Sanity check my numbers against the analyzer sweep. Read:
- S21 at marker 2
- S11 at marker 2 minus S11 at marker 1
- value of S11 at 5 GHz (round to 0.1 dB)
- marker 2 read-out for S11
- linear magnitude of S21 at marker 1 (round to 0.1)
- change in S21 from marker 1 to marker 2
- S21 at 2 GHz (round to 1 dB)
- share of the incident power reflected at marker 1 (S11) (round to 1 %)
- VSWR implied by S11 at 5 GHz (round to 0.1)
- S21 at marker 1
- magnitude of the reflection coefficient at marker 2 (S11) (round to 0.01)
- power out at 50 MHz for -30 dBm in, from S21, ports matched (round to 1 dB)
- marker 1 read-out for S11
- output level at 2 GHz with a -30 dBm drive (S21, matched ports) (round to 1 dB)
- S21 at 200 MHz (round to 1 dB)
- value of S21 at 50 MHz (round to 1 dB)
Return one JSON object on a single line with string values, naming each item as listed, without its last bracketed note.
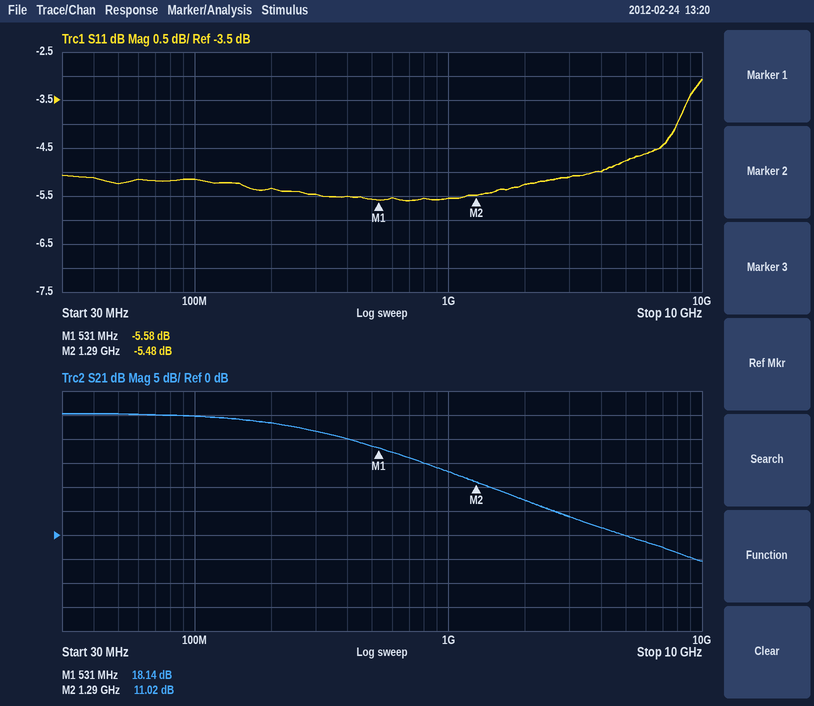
{"S21 at marker 2": "11.02 dB", "S11 at marker 2 minus S11 at marker 1": "0.10 dB", "value of S11 at 5 GHz": "-4.8 dB", "marker 2 read-out for S11": "-5.48 dB", "linear magnitude of S21 at marker 1": "8.1", "change in S21 from marker 1 to marker 2": "-7.12 dB", "S21 at 2 GHz": "7 dB", "share of the incident power reflected at marker 1 (S11)": "28 %", "VSWR implied by S11 at 5 GHz": "3.7", "S21 at marker 1": "18.14 dB", "magnitude of the reflection coefficient at marker 2 (S11)": "0.53", "power out at 50 MHz for -30 dBm in, from S21, ports matched": "-5 dBm", "marker 1 read-out for S11": "-5.58 dB", "output level at 2 GHz with a -30 dBm drive (S21, matched ports)": "-23 dBm", "S21 at 200 MHz": "23 dB", "value of S21 at 50 MHz": "25 dB"}
